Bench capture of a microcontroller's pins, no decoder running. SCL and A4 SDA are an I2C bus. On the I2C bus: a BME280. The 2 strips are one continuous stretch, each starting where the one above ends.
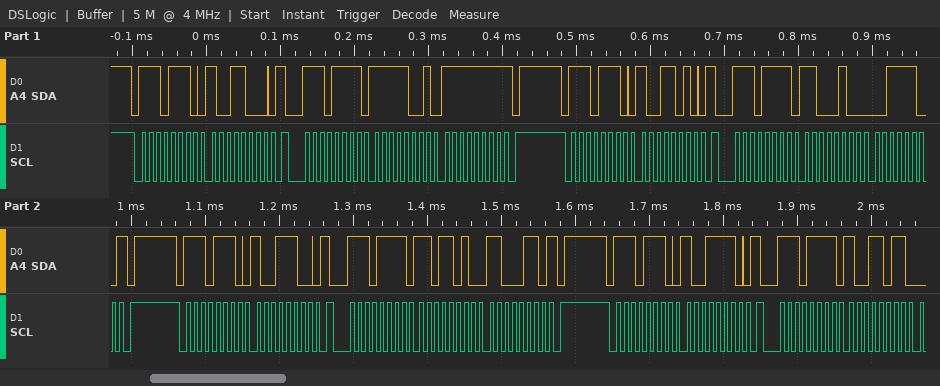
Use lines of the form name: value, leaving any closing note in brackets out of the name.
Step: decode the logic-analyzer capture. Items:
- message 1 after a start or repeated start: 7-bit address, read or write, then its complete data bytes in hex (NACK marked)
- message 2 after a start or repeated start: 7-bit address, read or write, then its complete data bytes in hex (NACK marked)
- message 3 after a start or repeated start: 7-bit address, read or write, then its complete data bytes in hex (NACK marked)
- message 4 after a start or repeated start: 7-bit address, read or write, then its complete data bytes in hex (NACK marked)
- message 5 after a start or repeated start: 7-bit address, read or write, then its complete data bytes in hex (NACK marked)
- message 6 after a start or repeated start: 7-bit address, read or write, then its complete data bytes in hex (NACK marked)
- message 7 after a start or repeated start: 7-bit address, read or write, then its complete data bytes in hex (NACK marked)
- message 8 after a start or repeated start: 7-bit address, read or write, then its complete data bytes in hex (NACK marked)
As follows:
message 1 after a start or repeated start: 7-bit address, read or write, then its complete data bytes in hex: 0x77 write: 98
message 2 after a start or repeated start: 7-bit address, read or write, then its complete data bytes in hex: 0x77 read: F9 FF NACK
message 3 after a start or repeated start: 7-bit address, read or write, then its complete data bytes in hex: 0x77 write: 9A
message 4 after a start or repeated start: 7-bit address, read or write, then its complete data bytes in hex: 0x77 read: C4 3C NACK
message 5 after a start or repeated start: 7-bit address, read or write, then its complete data bytes in hex: 0x77 write: 9C
message 6 after a start or repeated start: 7-bit address, read or write, then its complete data bytes in hex: 0x77 read: DA C6 NACK
message 7 after a start or repeated start: 7-bit address, read or write, then its complete data bytes in hex: 0x77 write: 9E
message 8 after a start or repeated start: 7-bit address, read or write, then its complete data bytes in hex: 0x77 read: 9B
